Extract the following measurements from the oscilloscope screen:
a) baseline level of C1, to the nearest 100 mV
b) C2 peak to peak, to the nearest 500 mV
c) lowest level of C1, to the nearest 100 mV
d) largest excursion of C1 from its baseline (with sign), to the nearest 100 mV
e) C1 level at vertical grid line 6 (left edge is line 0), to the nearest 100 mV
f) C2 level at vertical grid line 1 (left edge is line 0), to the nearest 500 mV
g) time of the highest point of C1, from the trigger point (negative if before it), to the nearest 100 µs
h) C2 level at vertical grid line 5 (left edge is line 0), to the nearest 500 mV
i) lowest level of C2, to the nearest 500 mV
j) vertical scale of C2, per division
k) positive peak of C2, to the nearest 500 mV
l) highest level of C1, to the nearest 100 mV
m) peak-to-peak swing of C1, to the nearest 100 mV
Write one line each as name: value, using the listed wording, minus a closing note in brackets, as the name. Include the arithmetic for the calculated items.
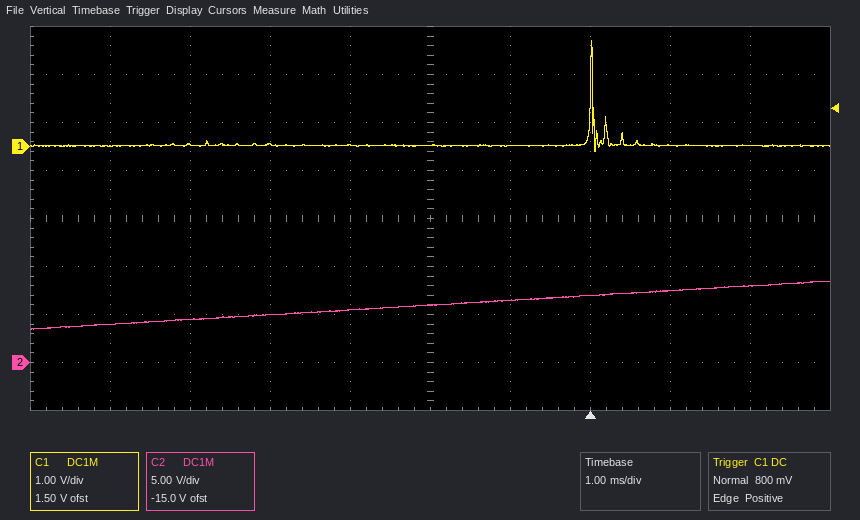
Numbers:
baseline level of C1, to the nearest 100 mV: 0.0 V
C2 peak to peak, to the nearest 500 mV: 8.5 V − (3.5 V) = 5.0 V
lowest level of C1, to the nearest 100 mV: -100 mV
largest excursion of C1 from its baseline (with sign), to the nearest 100 mV: 2.2 V − (0.0 V) = +2.2 V
C1 level at vertical grid line 6 (left edge is line 0), to the nearest 100 mV: 0.0 V
C2 level at vertical grid line 1 (left edge is line 0), to the nearest 500 mV: 4.0 V
time of the highest point of C1, from the trigger point (negative if before it), to the nearest 100 µs: 0.0 ms
C2 level at vertical grid line 5 (left edge is line 0), to the nearest 500 mV: 6.0 V
lowest level of C2, to the nearest 500 mV: 3.5 V
vertical scale of C2, per division: 5 V
positive peak of C2, to the nearest 500 mV: 8.5 V
highest level of C1, to the nearest 100 mV: 2.2 V
peak-to-peak swing of C1, to the nearest 100 mV: 2.2 V − (-100 mV) = 2.3 V
